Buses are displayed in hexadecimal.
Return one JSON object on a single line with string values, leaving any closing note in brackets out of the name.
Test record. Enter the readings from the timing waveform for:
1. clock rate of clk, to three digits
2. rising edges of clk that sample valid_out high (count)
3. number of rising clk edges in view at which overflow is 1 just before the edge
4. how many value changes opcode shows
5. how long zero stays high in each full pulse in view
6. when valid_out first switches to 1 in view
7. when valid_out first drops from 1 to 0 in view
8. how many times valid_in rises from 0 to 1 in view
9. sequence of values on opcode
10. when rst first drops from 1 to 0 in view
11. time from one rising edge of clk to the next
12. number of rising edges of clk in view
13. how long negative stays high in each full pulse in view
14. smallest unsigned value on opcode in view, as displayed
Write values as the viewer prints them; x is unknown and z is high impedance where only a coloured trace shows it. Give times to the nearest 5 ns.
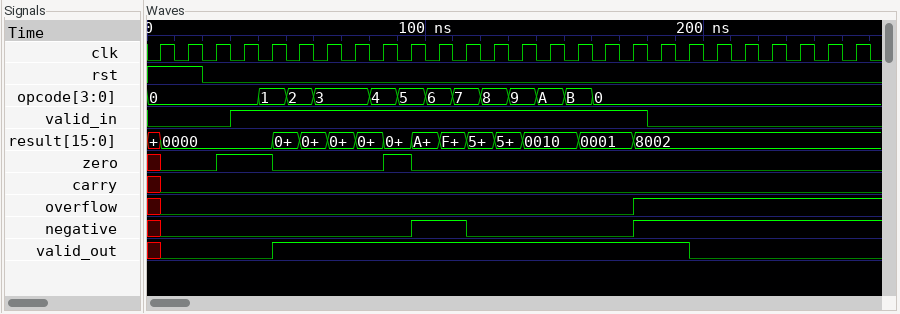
{"clock rate of clk, to three digits": "100 MHz", "rising edges of clk that sample valid_out high": "15", "number of rising clk edges in view at which overflow is 1 just before the edge": "8", "how many value changes opcode shows": "12", "how long zero stays high in each full pulse in view": "20 ns, 10 ns", "when valid_out first switches to 1 in view": "45 ns", "when valid_out first drops from 1 to 0 in view": "195 ns", "how many times valid_in rises from 0 to 1 in view": "1", "sequence of values on opcode": "0, 1, 2, 3, 4, 5, 6, 7, 8, 9, A, B, 0", "when rst first drops from 1 to 0 in view": "20 ns", "time from one rising edge of clk to the next": "10 ns", "number of rising edges of clk in view": "26", "how long negative stays high in each full pulse in view": "20 ns", "smallest unsigned value on opcode in view, as displayed": "0"}
